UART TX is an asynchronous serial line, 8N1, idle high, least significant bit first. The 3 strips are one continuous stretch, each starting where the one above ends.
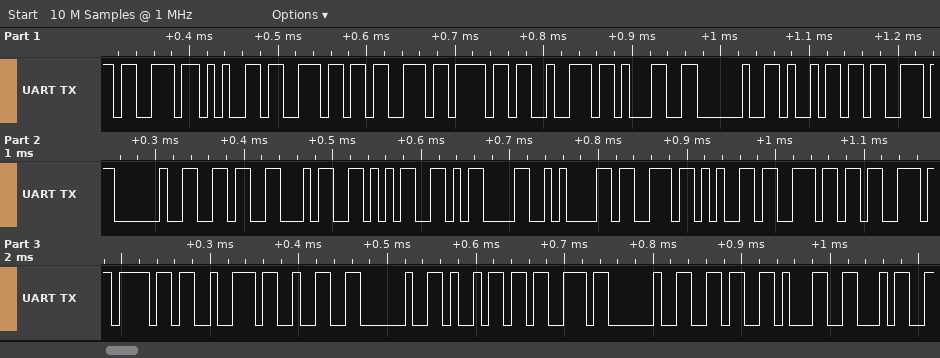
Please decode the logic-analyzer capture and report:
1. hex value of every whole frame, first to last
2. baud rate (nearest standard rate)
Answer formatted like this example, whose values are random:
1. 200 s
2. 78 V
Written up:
1. 73 65 6E 73 6F 72 31 20 69 73 20 36 34 35 0D 0A 73 65 6E 73 6F 72 32 20 69 73 20 36 31 34
2. 115200 baud
